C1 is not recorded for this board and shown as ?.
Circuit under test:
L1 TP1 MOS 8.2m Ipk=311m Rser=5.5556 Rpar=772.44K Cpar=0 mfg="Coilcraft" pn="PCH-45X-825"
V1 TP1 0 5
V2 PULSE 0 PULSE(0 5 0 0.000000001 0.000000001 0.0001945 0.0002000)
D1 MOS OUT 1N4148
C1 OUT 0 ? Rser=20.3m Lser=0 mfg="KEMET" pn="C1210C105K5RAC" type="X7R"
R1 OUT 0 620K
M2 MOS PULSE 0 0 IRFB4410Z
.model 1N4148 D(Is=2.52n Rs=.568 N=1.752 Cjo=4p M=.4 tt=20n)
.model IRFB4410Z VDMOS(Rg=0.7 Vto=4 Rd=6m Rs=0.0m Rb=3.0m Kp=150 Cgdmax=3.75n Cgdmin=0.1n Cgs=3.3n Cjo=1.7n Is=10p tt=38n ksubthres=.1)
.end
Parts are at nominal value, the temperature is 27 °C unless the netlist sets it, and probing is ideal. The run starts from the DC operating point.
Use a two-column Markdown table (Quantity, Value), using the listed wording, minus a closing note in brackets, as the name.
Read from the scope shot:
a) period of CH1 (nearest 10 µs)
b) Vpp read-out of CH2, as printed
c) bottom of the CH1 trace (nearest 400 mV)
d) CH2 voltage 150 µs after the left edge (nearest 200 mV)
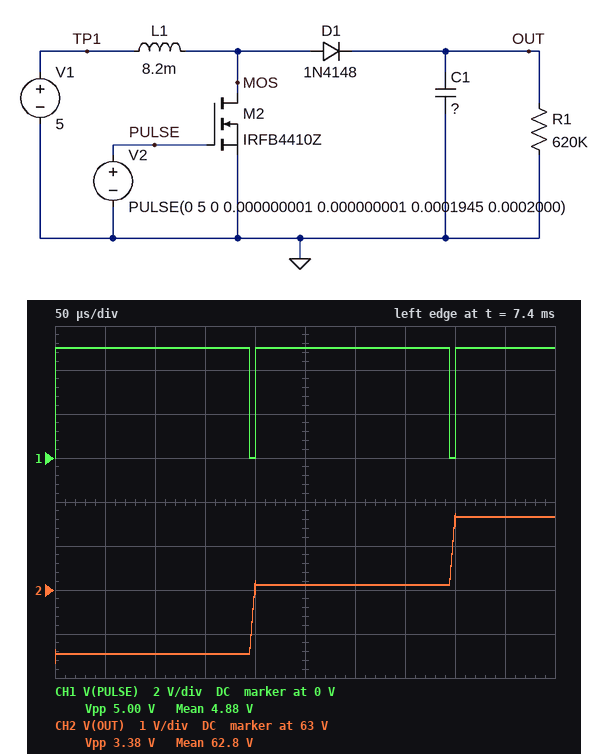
| Quantity | Value |
|---|---|
| period of CH1 | 200 µs |
| Vpp read-out of CH2, as printed | 3.38 V |
| bottom of the CH1 trace | 0 V |
| CH2 voltage 150 µs after the left edge | 61.6 V |
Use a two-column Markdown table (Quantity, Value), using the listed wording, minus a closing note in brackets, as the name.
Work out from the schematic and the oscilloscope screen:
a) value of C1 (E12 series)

| Quantity | Value |
|---|---|
| value of C1 | 2.2 µF |
